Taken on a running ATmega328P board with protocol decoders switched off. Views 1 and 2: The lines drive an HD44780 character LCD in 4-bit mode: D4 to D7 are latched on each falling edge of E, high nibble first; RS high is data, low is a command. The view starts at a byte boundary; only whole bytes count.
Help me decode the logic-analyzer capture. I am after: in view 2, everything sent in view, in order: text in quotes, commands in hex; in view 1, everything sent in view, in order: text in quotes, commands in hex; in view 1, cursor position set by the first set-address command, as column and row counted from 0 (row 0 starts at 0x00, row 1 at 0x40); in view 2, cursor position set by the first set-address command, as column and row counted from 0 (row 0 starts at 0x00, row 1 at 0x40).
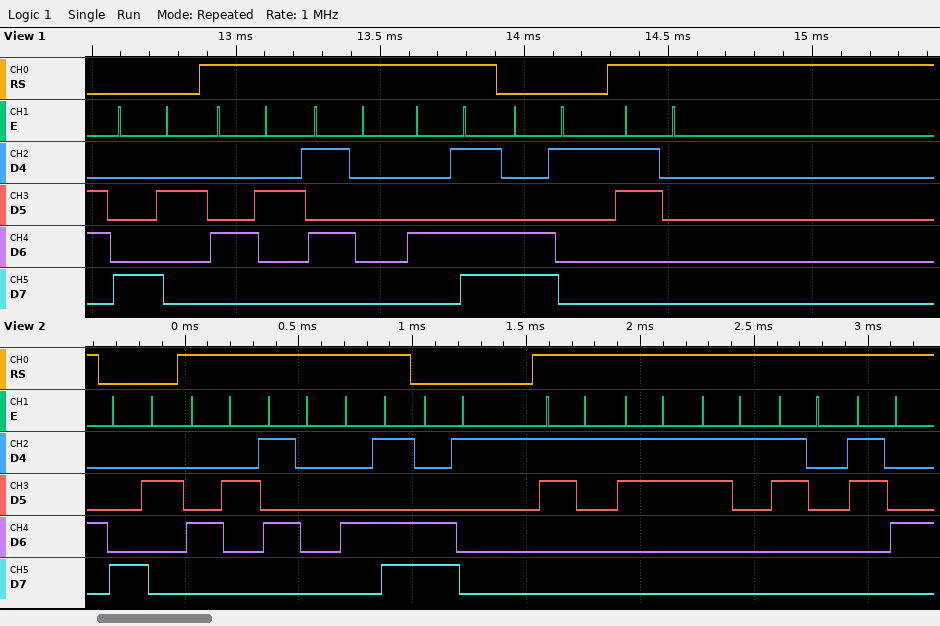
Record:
0x82 "BPM" 0xC1 "13104"
0x82 "BPM" 0xC1 "0"
column 2, row 0
column 2, row 0
